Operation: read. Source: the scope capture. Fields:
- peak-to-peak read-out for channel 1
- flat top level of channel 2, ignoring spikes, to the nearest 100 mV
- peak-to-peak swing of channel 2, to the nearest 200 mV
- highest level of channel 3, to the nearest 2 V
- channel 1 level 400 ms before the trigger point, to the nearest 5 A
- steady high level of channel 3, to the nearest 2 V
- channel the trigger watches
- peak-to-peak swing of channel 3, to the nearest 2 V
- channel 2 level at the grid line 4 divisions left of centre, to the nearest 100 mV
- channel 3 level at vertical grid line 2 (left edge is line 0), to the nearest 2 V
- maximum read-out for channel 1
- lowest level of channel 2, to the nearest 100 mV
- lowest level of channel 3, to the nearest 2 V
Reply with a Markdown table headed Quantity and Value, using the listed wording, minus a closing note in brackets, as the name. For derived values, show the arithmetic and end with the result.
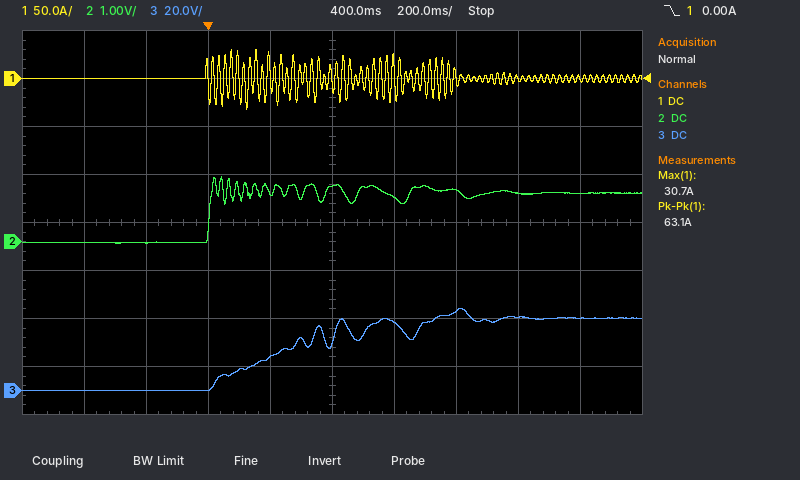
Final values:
| Quantity | Value |
|---|---|
| peak-to-peak read-out for channel 1 | 63.1 A |
| flat top level of channel 2, ignoring spikes, to the nearest 100 mV | 1.0 V |
| peak-to-peak swing of channel 2, to the nearest 200 mV | 1.4 V |
| highest level of channel 3, to the nearest 2 V | 34 V |
| channel 1 level 400 ms before the trigger point, to the nearest 5 A | 0 A |
| steady high level of channel 3, to the nearest 2 V | 30 V |
| channel the trigger watches | channel 1 |
| peak-to-peak swing of channel 3, to the nearest 2 V | 34 V − (0 V) = 34 V |
| channel 2 level at the grid line 4 divisions left of centre, to the nearest 100 mV | 0.0 V |
| channel 3 level at vertical grid line 2 (left edge is line 0), to the nearest 2 V | 0 V |
| maximum read-out for channel 1 | 30.7 A |
| lowest level of channel 2, to the nearest 100 mV | 0.0 V |
| lowest level of channel 3, to the nearest 2 V | 0 V |
